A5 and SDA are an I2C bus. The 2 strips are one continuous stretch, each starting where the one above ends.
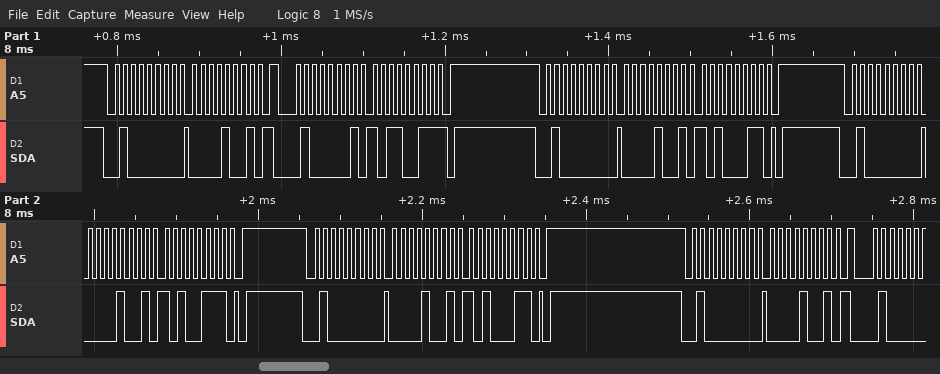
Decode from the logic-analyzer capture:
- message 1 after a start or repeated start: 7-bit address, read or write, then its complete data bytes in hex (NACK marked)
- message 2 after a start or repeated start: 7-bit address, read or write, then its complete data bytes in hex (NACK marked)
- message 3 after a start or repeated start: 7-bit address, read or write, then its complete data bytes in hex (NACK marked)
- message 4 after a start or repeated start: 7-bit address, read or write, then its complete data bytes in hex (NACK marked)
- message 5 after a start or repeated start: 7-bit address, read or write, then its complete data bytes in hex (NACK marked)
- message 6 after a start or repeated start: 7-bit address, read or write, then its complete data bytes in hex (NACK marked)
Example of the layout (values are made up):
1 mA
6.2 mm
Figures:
0x20 write: 09
0x20 read: B3 NACK
0x20 write: 09 A3
0x20 write: 09 A7
0x20 write: 09 A3
0x20 write: 09
